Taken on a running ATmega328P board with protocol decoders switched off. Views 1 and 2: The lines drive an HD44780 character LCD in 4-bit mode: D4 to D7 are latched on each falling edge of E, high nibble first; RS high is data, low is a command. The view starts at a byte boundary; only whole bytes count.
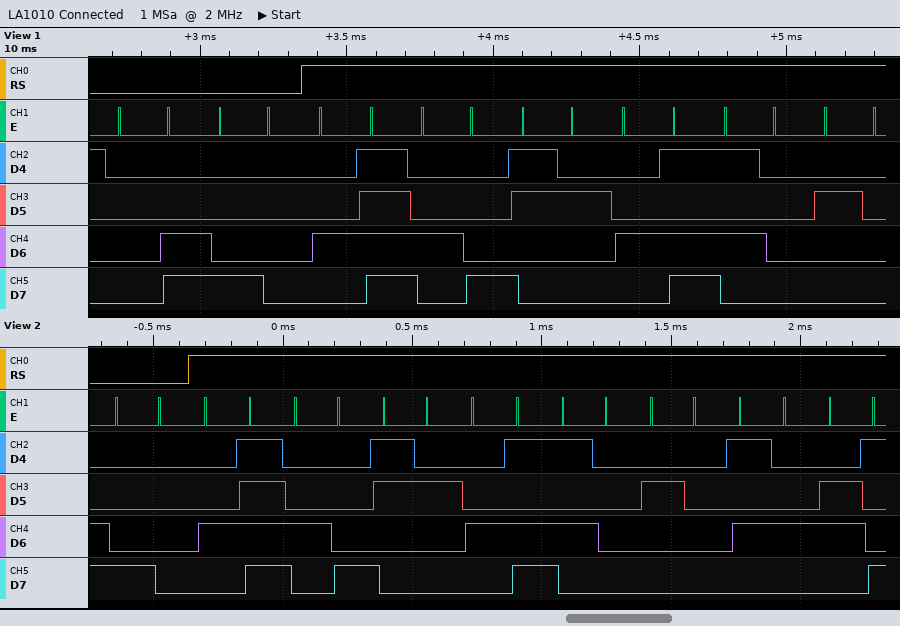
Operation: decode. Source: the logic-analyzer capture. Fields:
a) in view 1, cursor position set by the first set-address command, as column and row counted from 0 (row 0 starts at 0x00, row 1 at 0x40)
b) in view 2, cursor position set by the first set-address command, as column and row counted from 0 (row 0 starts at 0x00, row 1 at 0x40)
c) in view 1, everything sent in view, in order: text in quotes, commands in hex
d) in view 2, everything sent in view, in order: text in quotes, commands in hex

column 0, row 0
column 0, row 0
0x0C 0x80 "OH2MP "
0x80 "OH2MP Ti"
